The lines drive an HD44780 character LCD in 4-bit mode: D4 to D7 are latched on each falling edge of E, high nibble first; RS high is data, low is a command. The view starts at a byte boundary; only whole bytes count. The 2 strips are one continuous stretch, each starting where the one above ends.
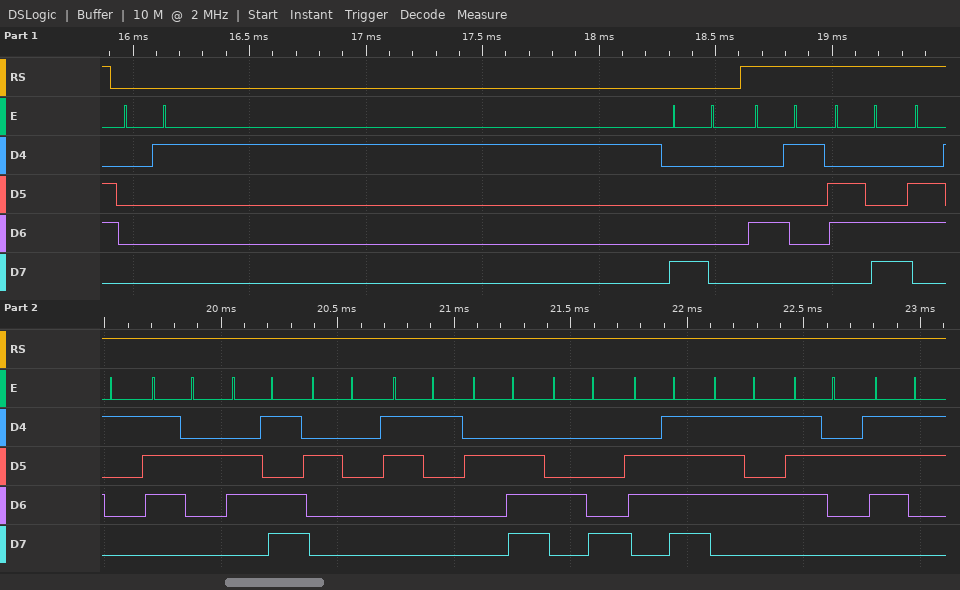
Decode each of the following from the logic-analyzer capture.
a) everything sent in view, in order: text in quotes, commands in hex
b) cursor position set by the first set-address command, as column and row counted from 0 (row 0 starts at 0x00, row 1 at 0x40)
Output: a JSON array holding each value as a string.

["0x01 0x80 \"Alarm 1.Hours\"", "column 0, row 0"]
